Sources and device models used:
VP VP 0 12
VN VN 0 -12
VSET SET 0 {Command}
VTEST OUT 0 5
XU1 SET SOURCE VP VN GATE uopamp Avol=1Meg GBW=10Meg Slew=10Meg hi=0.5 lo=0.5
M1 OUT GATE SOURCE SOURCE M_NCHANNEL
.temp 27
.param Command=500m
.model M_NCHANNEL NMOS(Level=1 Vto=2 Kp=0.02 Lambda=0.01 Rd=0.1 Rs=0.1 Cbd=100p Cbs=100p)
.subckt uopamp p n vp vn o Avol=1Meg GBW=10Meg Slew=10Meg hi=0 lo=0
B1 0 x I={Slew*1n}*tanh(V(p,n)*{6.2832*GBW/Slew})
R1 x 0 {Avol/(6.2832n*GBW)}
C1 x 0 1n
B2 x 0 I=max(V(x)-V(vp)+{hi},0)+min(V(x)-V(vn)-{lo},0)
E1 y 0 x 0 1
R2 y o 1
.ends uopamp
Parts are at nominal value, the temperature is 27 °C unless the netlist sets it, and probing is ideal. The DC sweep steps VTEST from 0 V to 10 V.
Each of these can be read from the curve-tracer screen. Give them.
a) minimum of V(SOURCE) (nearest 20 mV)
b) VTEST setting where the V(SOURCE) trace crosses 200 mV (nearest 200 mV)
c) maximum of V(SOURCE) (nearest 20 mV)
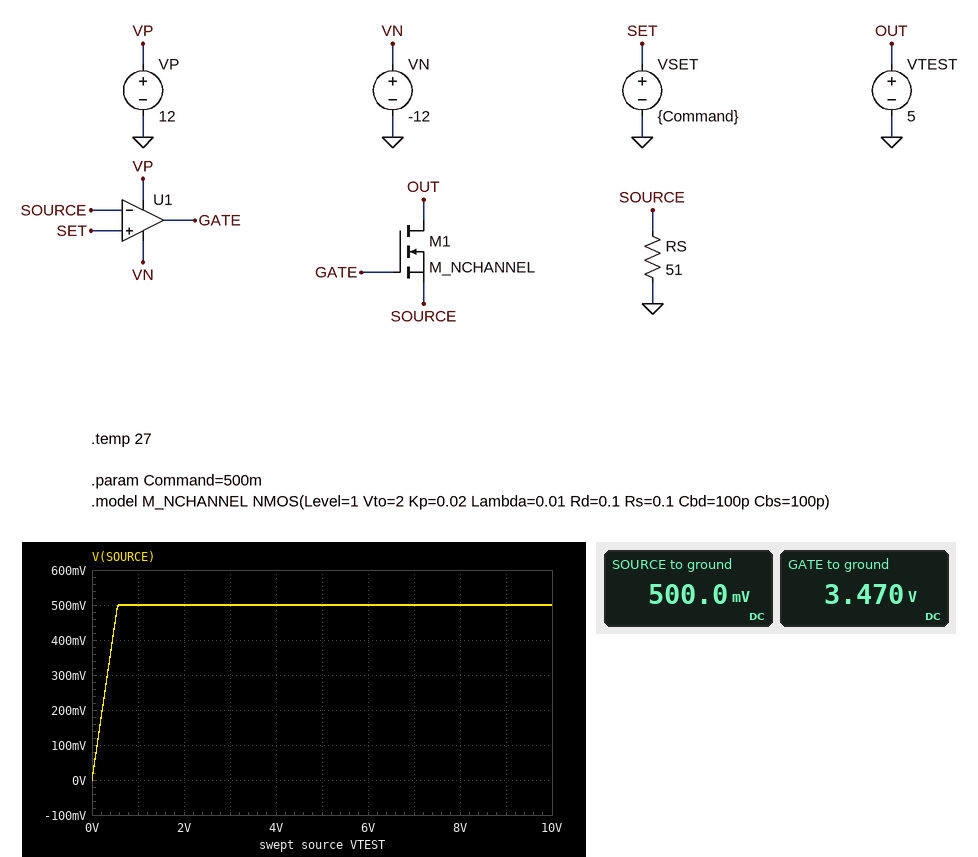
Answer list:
0 V
200 mV
500 mV
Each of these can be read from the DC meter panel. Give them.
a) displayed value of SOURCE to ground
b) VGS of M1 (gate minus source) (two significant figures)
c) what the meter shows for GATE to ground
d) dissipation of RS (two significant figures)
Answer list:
500.0 mV
3.0 V
3.470 V
4.9 mW
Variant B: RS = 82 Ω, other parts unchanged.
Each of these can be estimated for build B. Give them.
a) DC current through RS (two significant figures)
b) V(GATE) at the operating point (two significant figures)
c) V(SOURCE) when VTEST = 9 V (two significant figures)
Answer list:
6.1 mA
3.3 V
500 mV
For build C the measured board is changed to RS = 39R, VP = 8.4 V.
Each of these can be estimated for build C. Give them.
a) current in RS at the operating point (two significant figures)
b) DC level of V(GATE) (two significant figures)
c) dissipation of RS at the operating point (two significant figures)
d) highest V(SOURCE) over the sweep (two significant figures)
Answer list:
13 mA
3.6 V
6.4 mW
500 mV
